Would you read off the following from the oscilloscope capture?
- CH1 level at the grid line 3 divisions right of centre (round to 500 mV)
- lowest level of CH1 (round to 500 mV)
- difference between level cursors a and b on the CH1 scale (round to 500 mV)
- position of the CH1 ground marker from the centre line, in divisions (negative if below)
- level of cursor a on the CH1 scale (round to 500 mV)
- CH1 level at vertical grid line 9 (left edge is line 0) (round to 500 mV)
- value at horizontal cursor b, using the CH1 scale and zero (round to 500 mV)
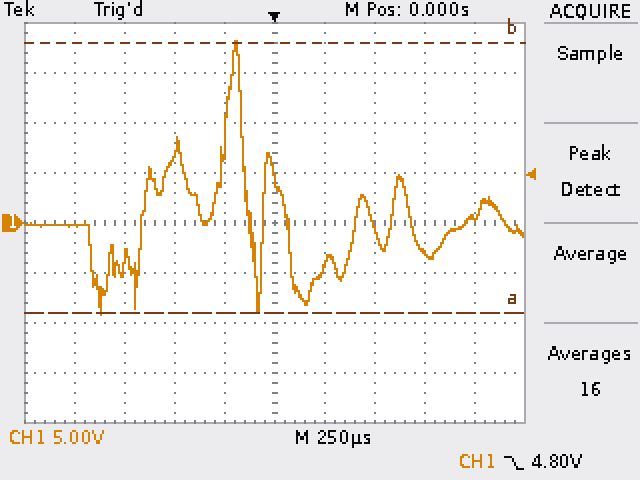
-3.0 V
-9.0 V
27.0 V
0.0 div
-9.0 V
500 mV
18.0 V
